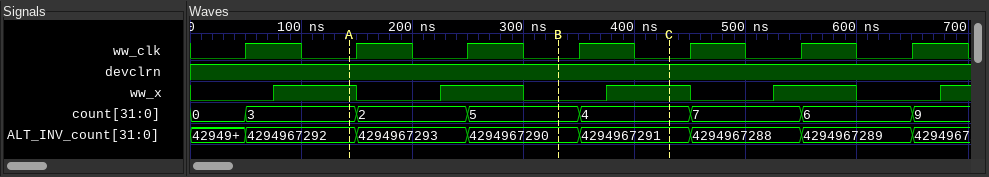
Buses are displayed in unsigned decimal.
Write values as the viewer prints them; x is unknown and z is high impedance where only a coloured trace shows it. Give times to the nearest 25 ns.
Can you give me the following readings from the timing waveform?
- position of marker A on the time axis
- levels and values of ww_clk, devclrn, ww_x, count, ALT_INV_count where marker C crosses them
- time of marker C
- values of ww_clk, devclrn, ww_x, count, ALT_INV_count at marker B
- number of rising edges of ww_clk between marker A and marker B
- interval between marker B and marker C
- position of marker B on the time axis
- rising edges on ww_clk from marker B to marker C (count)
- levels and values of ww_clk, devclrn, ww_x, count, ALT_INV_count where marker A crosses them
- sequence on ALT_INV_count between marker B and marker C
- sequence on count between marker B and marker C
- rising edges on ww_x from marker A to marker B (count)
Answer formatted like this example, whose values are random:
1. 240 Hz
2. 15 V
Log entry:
1. 150 ns
2. ww_clk=0, devclrn=1, ww_x=1, count=4, ALT_INV_count=4294967291
3. 425 ns
4. ww_clk=0, devclrn=1, ww_x=0, count=5, ALT_INV_count=4294967290
5. 2
6. 100 ns
7. 325 ns
8. 1
9. ww_clk=0, devclrn=1, ww_x=1, count=3, ALT_INV_count=4294967292
10. 4294967290, 4294967291
11. 5, 4
12. 1
